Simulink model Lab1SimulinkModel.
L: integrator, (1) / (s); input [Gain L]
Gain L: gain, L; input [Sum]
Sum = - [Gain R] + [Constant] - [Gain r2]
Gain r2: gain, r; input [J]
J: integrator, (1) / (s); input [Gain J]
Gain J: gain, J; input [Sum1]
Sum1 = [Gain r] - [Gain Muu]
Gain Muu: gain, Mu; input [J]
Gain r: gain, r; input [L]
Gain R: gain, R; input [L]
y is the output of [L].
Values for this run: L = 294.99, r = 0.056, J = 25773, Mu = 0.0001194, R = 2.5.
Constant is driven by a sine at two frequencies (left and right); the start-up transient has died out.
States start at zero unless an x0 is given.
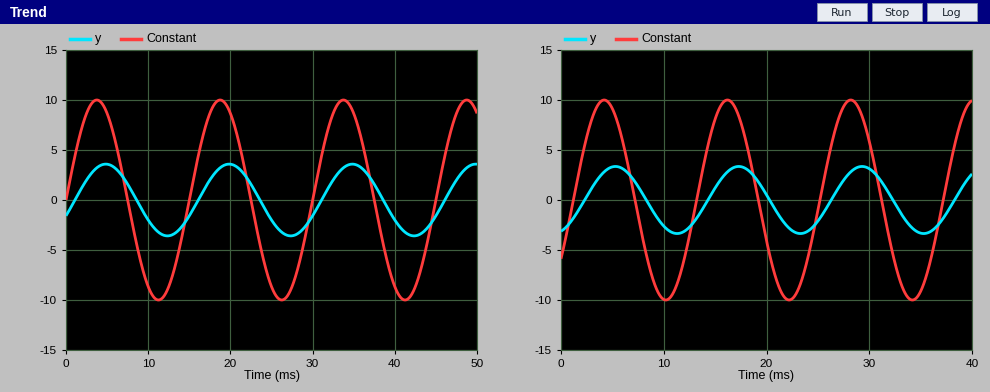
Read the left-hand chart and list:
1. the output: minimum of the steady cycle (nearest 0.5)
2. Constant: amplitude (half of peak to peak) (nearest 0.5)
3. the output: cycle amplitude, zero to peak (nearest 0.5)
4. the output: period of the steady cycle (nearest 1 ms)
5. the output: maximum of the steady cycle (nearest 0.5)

-3.5
10.0
3.5
15 ms
3.5
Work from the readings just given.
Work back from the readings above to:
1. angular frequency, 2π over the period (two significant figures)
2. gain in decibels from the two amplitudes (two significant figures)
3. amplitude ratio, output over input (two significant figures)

0.42 rad/ms
-9.1 dB
0.35
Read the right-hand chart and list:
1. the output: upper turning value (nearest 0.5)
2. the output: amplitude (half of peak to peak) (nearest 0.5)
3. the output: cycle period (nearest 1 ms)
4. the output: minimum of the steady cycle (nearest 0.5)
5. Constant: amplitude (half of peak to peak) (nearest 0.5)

3.5
3.5
12 ms
-3.5
10.0
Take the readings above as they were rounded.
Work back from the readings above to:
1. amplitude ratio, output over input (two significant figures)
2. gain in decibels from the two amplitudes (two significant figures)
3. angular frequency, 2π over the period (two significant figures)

0.35
-9.1 dB
0.52 rad/ms
